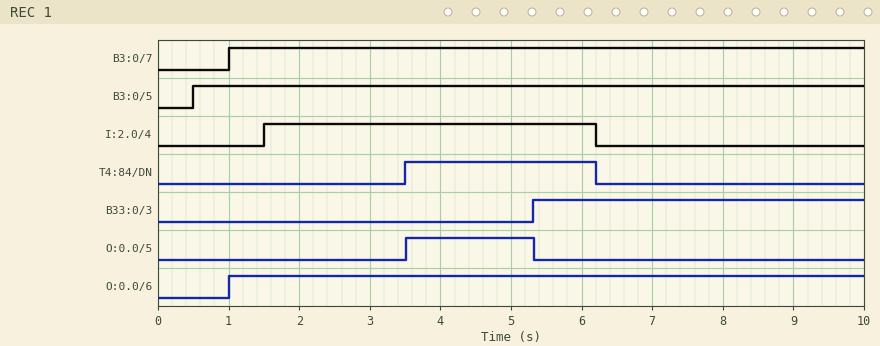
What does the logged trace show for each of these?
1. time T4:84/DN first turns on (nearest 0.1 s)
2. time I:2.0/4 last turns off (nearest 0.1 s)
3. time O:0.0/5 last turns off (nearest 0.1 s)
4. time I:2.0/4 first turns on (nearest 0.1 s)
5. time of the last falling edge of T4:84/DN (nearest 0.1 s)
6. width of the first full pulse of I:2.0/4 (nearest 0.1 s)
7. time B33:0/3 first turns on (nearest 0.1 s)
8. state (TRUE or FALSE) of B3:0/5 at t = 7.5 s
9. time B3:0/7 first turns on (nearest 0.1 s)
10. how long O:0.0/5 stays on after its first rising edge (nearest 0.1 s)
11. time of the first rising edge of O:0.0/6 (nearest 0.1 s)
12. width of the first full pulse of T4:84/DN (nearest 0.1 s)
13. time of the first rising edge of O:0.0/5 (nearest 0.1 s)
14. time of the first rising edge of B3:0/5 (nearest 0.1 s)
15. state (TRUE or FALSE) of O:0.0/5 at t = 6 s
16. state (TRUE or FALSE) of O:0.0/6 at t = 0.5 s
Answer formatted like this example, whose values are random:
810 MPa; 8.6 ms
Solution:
3.5 s; 6.2 s; 5.3 s; 1.5 s; 6.2 s; 4.7 s; 5.3 s; TRUE; 1.0 s; 1.8 s; 1.0 s; 2.7 s; 3.5 s; 0.5 s; FALSE; FALSE
